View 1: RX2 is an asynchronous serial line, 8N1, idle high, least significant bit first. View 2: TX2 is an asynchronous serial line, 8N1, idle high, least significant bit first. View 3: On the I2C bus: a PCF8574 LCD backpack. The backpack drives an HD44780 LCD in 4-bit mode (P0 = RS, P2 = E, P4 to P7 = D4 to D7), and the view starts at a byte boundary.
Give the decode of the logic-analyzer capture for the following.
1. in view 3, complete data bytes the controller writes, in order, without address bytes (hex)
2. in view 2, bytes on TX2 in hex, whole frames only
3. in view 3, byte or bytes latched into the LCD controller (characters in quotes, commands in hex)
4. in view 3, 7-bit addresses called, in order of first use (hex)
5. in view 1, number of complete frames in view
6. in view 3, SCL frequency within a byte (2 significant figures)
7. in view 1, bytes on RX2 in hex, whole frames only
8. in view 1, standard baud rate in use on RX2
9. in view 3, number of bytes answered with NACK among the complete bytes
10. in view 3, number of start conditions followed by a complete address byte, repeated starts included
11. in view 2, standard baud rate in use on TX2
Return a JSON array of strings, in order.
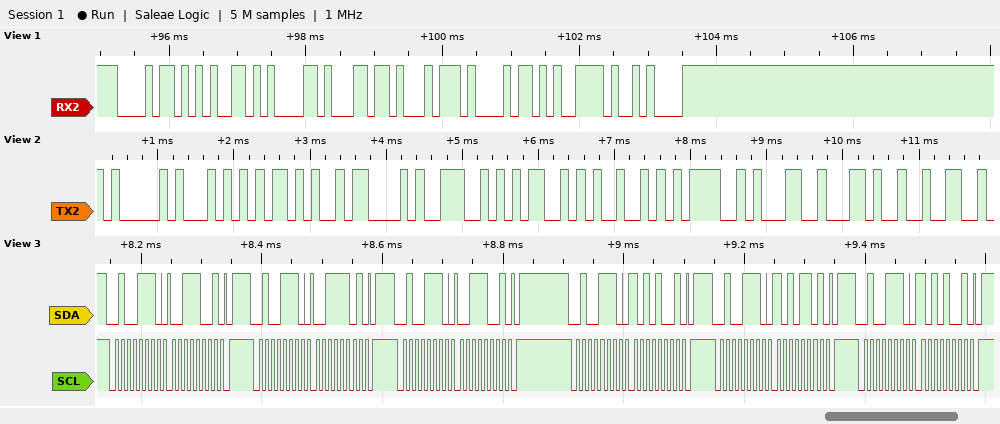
["39 3D 39 A9 AD A9", "0x41 0x54 0x2B 0x43 0x4E 0x4D 0x49 0x3D 0x31 0x2C 0x32", "':'", "0x27", "8", "100 kHz", "0x68 0x65 0x61 0x6C 0x74 0x68 0x79 0x0A", "9600 baud", "0", "6", "9600 baud"]
